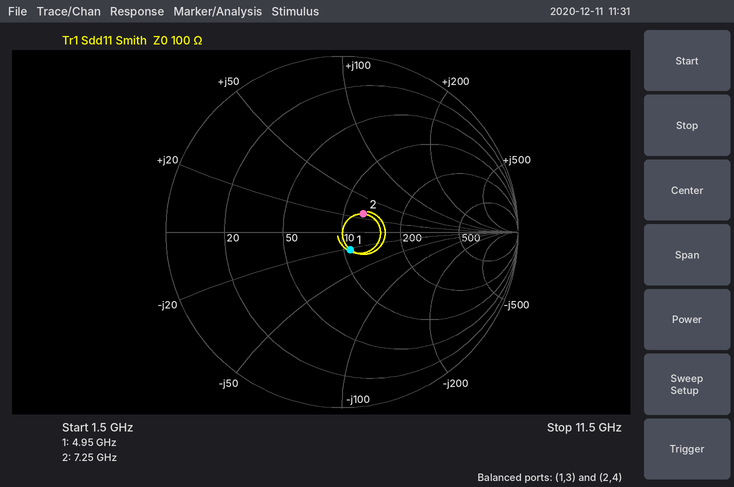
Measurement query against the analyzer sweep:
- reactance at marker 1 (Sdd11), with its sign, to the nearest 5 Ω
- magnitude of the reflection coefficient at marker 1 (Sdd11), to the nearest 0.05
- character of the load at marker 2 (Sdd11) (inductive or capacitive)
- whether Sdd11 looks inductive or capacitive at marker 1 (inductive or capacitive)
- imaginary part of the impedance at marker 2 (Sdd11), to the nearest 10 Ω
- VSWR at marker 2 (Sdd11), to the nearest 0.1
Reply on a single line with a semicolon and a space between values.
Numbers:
-20 Ω; 0.10; inductive; capacitive; +30 Ω; 1.4
